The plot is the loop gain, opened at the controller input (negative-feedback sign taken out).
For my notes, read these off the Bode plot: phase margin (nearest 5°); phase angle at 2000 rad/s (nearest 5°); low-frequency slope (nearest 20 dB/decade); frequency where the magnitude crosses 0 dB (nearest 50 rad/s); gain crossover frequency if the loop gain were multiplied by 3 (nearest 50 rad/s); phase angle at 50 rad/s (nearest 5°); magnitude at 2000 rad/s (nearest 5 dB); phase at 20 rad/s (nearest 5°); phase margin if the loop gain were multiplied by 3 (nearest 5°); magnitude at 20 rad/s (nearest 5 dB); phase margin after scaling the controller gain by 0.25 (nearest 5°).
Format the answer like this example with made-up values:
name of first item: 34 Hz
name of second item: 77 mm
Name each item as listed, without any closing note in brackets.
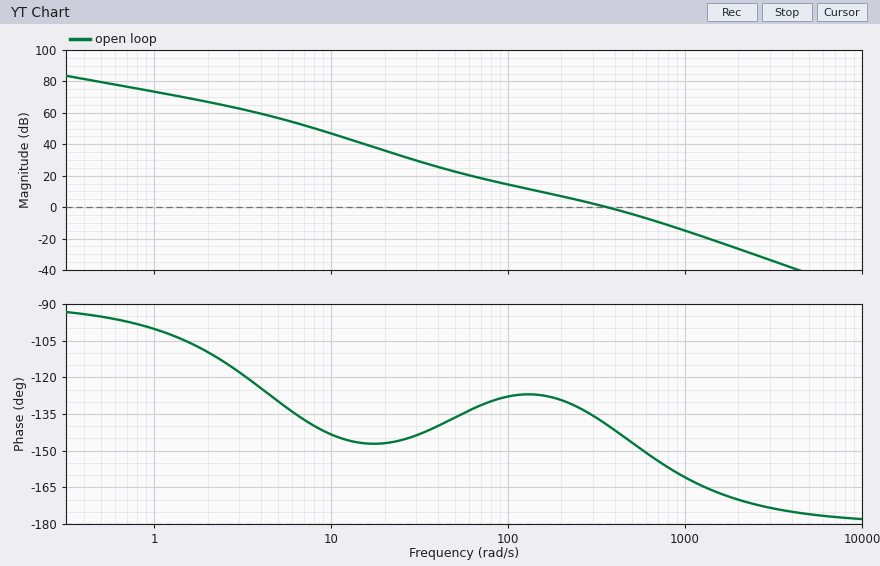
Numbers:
phase margin: 40°
phase angle at 2000 rad/s: -170°
low-frequency slope: -20 dB/decade
frequency where the magnitude crosses 0 dB: 350 rad/s
gain crossover frequency if the loop gain were multiplied by 3: 700 rad/s
phase angle at 50 rad/s: -135°
magnitude at 2000 rad/s: -25 dB
phase at 20 rad/s: -145°
phase margin if the loop gain were multiplied by 3: 25°
magnitude at 20 rad/s: 35 dB
phase margin after scaling the controller gain by 0.25: 55°
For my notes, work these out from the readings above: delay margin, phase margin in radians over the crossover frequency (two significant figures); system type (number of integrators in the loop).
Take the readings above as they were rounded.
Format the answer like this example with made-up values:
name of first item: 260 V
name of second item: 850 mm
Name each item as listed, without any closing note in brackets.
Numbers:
delay margin, phase margin in radians over the crossover frequency: 0.0020 s
system type: 1
